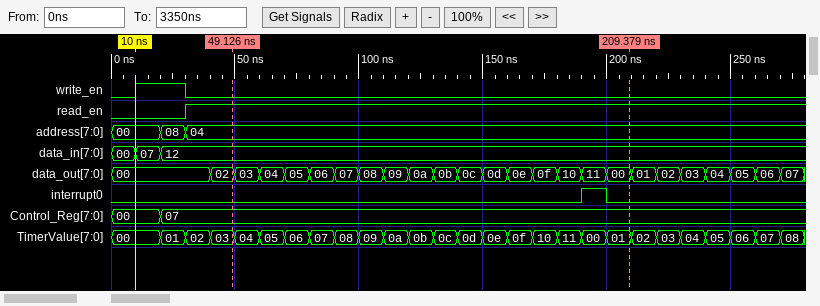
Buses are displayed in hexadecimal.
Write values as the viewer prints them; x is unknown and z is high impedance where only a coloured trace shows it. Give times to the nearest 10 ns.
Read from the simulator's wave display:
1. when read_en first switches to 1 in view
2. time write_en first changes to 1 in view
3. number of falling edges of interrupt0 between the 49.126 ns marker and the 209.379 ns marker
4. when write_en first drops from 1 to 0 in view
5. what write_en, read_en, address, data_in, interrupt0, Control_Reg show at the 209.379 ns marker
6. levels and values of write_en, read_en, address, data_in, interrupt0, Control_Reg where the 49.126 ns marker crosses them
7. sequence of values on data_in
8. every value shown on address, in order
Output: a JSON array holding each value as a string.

["30 ns", "10 ns", "1", "30 ns", "write_en=0, read_en=1, address=04, data_in=12, interrupt0=0, Control_Reg=07", "write_en=0, read_en=1, address=04, data_in=12, interrupt0=0, Control_Reg=07", "00, 07, 12", "00, 08, 04"]
